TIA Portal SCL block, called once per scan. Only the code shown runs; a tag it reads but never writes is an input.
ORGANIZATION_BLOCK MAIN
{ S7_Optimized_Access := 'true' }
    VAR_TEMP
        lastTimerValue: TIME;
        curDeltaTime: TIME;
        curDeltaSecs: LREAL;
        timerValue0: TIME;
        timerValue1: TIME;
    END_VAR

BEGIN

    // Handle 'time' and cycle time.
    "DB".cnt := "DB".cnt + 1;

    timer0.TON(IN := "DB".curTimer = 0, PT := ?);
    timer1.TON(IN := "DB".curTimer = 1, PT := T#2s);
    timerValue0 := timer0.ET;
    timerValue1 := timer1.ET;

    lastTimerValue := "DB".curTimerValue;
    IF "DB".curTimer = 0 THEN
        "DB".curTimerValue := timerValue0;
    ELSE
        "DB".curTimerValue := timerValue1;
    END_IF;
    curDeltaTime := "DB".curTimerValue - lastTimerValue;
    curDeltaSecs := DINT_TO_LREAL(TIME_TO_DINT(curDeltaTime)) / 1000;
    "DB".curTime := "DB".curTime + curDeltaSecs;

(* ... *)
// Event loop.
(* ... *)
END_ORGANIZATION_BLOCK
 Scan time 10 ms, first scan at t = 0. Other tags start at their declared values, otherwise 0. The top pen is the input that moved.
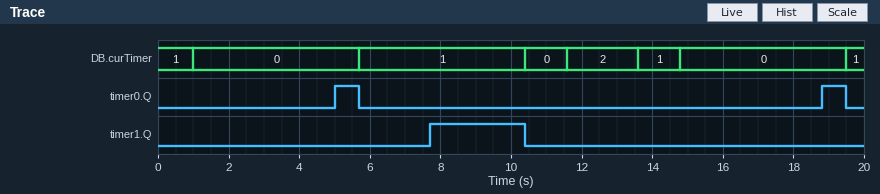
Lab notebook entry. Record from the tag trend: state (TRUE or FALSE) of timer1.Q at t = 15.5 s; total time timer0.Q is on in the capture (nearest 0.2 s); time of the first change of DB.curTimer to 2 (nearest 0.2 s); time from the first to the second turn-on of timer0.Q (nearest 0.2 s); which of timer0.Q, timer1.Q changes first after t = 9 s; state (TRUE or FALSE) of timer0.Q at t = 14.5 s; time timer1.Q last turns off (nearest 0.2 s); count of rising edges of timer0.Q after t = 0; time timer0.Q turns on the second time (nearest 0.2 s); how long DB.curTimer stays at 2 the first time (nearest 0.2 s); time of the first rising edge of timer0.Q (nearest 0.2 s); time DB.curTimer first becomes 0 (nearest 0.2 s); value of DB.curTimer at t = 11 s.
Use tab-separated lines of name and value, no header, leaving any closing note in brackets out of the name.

state (TRUE or FALSE) of timer1.Q at t = 15.5 s	FALSE
total time timer0.Q is on in the capture	1.4 s
time of the first change of DB.curTimer to 2	11.6 s
time from the first to the second turn-on of timer0.Q	13.8 s
which of timer0.Q, timer1.Q changes first after t = 9 s	timer1.Q
state (TRUE or FALSE) of timer0.Q at t = 14.5 s	FALSE
time timer1.Q last turns off	10.4 s
count of rising edges of timer0.Q after t = 0	2
time timer0.Q turns on the second time	18.8 s
how long DB.curTimer stays at 2 the first time	2.0 s
time of the first rising edge of timer0.Q	5.0 s
time DB.curTimer first becomes 0	1.0 s
value of DB.curTimer at t = 11 s	0
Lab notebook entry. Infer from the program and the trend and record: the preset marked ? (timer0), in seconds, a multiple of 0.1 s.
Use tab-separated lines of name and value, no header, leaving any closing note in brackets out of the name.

the preset marked ? (timer0), in seconds, a multiple of 0.1 s	4.0 s
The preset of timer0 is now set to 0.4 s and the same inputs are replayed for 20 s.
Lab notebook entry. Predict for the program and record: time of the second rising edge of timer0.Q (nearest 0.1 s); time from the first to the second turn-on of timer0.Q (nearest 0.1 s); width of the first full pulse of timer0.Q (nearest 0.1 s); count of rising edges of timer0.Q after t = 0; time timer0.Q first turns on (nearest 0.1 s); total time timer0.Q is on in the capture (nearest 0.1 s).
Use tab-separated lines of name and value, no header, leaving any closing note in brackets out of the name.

time of the second rising edge of timer0.Q	10.8 s
time from the first to the second turn-on of timer0.Q	9.4 s
width of the first full pulse of timer0.Q	4.3 s
count of rising edges of timer0.Q after t = 0	3
time timer0.Q first turns on	1.4 s
total time timer0.Q is on in the capture	9.4 s
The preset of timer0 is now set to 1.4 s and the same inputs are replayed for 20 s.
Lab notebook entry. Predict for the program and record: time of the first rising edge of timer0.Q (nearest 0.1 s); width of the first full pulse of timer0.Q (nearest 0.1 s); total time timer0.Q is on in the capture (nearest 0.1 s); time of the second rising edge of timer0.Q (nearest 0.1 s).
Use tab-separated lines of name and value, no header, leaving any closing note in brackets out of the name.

time of the first rising edge of timer0.Q	2.4 s
width of the first full pulse of timer0.Q	3.3 s
total time timer0.Q is on in the capture	6.6 s
time of the second rising edge of timer0.Q	16.2 s
